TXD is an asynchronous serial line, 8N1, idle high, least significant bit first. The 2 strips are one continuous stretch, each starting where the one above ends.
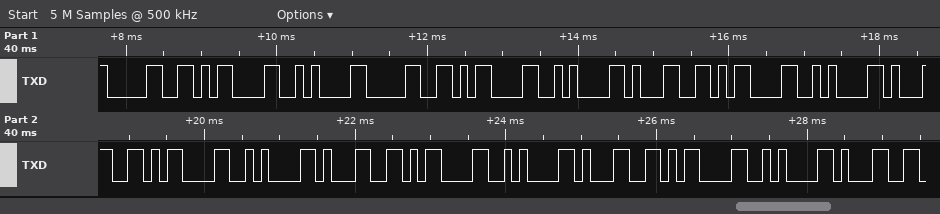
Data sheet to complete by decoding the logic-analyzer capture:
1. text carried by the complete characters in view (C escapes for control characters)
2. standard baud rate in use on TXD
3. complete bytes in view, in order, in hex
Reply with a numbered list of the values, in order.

1. "0\r\n0\r\n1\r\n1\r\n1\r\n1\r\n1"
2. 9600 baud
3. 30 0D 0A 30 0D 0A 31 0D 0A 31 0D 0A 31 0D 0A 31 0D 0A 31
